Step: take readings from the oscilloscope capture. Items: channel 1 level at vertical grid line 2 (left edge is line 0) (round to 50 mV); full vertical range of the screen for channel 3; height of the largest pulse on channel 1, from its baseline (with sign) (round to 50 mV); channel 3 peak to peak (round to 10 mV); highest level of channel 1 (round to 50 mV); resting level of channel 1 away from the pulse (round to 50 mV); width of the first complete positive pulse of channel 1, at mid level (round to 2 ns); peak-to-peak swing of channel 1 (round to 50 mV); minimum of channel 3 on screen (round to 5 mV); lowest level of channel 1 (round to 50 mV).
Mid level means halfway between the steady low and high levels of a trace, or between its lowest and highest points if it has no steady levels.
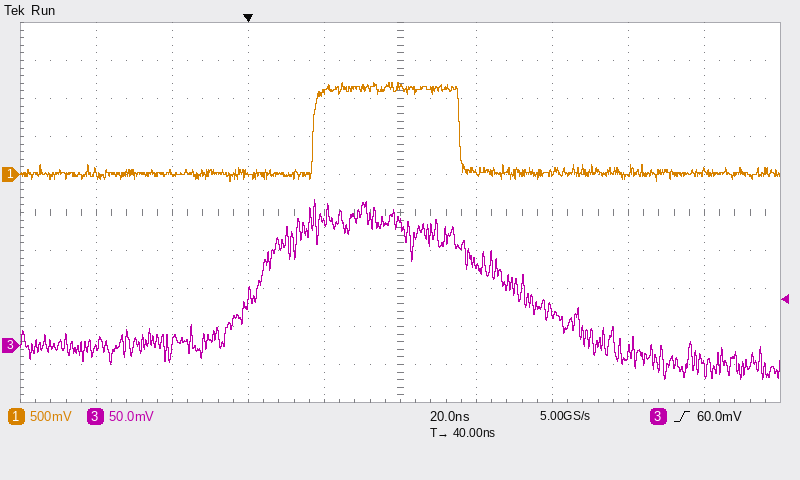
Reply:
0 mV
500 mV
+1.20 V
240 mV
1.20 V
0 mV
38 ns
1.30 V
-45 mV
-100 mV
